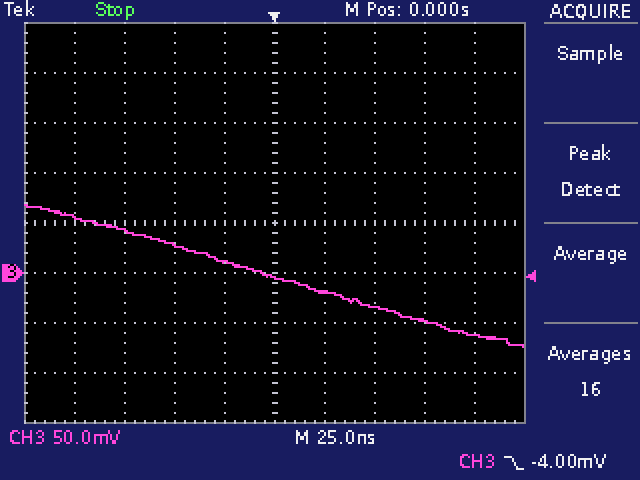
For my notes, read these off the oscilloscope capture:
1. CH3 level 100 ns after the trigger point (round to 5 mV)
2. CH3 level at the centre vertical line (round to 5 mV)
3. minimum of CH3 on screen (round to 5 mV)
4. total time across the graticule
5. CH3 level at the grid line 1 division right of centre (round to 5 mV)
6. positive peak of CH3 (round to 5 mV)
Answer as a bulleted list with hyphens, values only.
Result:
- -60 mV
- -5 mV
- -75 mV
- 250 ns
- -20 mV
- 70 mV
